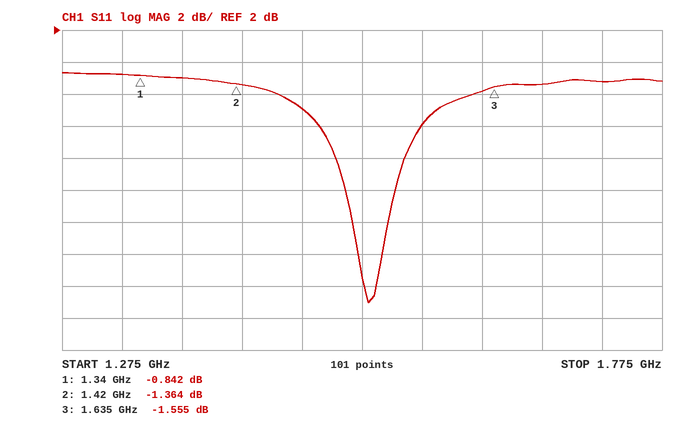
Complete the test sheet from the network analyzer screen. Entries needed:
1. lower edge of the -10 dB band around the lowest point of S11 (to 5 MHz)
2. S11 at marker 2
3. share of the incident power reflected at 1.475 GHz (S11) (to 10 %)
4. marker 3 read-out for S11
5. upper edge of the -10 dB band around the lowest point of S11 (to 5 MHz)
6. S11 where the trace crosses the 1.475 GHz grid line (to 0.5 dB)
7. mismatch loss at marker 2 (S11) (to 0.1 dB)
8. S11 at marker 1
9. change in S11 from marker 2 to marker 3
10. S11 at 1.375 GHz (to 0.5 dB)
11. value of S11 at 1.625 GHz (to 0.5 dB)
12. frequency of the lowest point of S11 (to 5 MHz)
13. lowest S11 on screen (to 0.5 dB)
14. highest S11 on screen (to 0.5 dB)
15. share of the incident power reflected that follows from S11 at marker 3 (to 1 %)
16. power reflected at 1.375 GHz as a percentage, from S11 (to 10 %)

1.515 GHz
-1.364 dB
50 %
-1.555 dB
1.545 GHz
-3.0 dB
5.7 dB
-0.842 dB
-0.191 dB
-1.0 dB
-2.0 dB
1.530 GHz
-15.0 dB
-0.5 dB
70 %
80 %
